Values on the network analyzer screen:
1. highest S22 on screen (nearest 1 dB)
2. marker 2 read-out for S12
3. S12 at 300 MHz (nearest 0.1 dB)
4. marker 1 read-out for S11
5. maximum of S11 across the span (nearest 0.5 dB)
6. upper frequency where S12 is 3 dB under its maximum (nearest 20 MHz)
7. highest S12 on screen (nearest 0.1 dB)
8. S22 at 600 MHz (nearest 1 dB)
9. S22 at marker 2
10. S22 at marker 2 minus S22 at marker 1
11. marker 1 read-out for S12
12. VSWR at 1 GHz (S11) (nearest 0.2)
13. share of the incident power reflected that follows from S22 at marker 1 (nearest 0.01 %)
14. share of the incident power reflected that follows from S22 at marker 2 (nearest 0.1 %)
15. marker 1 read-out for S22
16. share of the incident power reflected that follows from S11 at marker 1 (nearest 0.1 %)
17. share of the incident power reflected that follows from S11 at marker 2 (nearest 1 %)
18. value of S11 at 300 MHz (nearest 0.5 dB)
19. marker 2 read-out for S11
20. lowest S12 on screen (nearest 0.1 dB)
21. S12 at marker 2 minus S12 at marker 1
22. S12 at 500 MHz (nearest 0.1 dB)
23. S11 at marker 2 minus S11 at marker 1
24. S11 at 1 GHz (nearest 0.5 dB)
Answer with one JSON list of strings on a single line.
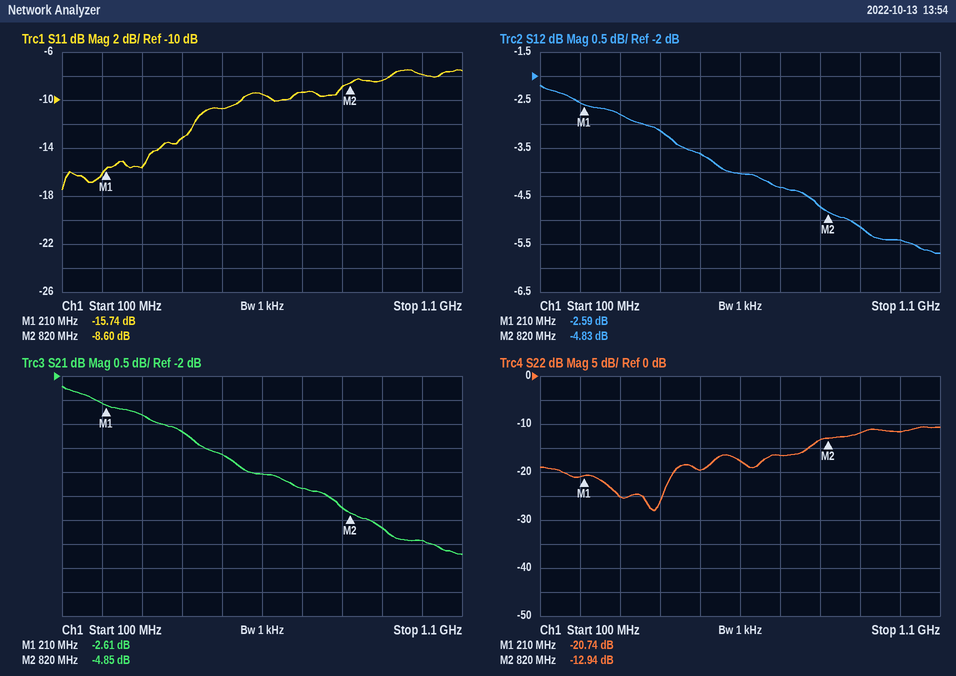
["-11 dB", "-4.83 dB", "-2.8 dB", "-15.74 dB", "-7.5 dB", "900 MHz", "-2.2 dB", "-18 dB", "-12.94 dB", "7.80 dB", "-2.59 dB", "2.4", "0.84 %", "5.1 %", "-20.74 dB", "2.7 %", "14 %", "-15.5 dB", "-8.60 dB", "-5.7 dB", "-2.24 dB", "-3.6 dB", "7.14 dB", "-8.0 dB"]
